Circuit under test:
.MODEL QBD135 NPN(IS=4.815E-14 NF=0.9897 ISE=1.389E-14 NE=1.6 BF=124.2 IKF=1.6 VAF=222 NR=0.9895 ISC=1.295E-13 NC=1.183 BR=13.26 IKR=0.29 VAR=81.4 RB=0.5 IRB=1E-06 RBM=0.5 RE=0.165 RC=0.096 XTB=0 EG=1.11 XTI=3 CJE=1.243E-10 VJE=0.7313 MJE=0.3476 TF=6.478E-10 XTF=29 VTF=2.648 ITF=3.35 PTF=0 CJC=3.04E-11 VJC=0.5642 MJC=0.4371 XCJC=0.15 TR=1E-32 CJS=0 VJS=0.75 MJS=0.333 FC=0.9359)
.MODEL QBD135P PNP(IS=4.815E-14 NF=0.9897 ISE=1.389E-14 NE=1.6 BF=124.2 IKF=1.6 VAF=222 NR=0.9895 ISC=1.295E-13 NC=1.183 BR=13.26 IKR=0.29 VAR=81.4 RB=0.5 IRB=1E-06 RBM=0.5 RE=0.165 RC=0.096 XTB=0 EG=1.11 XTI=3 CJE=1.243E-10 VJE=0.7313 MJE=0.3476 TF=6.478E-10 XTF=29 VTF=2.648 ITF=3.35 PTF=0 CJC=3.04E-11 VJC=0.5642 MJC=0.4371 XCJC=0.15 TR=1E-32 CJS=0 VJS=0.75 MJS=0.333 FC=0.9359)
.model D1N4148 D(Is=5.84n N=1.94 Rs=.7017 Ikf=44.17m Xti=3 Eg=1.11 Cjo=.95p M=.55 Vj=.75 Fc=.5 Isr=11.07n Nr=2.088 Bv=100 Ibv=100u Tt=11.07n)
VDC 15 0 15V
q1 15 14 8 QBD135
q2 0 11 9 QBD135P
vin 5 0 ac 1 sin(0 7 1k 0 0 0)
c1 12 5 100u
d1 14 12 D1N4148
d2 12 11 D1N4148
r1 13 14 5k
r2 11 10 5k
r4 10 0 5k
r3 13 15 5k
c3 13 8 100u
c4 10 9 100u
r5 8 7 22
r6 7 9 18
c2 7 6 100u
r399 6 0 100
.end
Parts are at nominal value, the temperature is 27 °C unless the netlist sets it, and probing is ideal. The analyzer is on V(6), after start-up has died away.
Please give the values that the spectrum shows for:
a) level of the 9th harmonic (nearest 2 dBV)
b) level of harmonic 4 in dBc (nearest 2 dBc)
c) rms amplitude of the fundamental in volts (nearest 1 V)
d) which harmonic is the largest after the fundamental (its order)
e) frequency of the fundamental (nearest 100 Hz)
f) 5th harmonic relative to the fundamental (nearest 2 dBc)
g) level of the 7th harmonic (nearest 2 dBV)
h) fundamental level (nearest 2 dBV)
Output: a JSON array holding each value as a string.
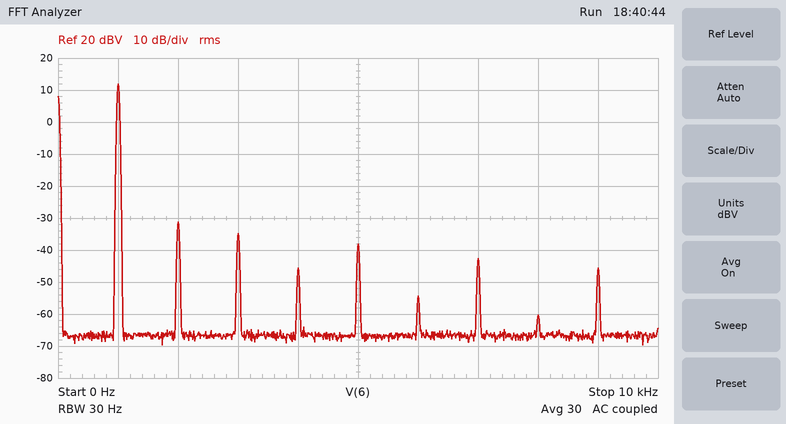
["-46 dBV", "-58 dBc", "4 V", "2", "1.0 kHz", "-50 dBc", "-42 dBV", "12 dBV"]
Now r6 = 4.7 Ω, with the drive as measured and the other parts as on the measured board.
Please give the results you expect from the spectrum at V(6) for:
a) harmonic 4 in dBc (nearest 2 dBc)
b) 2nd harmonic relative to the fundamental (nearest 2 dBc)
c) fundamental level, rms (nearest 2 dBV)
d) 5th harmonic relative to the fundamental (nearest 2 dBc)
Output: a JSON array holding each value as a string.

["-44 dBc", "-30 dBc", "12 dBV", "-48 dBc"]
